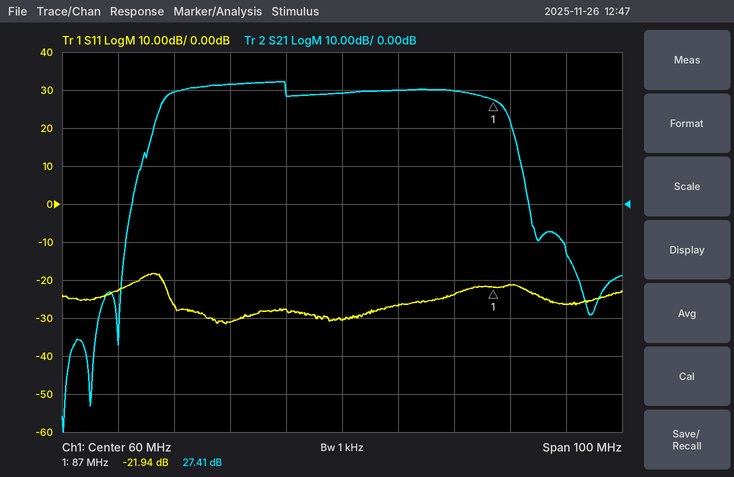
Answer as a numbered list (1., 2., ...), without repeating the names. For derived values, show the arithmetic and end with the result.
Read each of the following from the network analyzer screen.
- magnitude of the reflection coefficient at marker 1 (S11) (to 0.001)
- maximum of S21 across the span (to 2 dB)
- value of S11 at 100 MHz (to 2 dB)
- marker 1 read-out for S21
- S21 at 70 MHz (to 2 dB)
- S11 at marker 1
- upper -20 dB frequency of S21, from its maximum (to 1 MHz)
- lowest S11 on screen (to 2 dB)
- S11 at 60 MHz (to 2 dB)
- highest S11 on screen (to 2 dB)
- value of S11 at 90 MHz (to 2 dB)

1. 10^(-21.94/20) ≈ 0.080
2. 32 dB
3. -26 dB
4. 27.41 dB
5. 30 dB
6. -21.94 dB
7. 92 MHz
8. -32 dB
9. -30 dB
10. -18 dB
11. -22 dB
